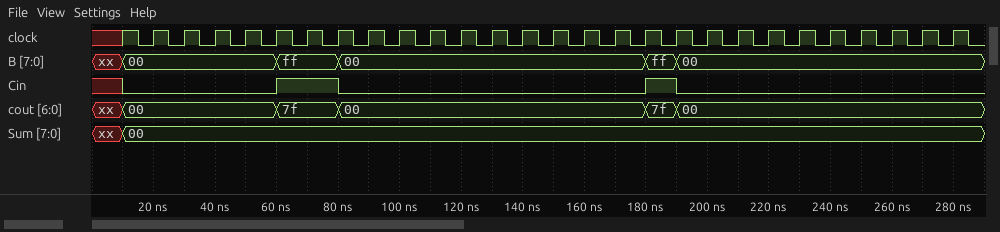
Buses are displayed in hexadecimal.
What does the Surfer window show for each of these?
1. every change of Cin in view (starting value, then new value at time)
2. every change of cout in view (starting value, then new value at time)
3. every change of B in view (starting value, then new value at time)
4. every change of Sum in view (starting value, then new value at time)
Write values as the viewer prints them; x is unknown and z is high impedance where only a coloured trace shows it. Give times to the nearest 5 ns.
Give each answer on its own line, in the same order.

x, 0 at 10 ns, 1 at 60 ns, 0 at 80 ns, 1 at 180 ns, 0 at 190 ns
xx, 00 at 10 ns, 7f at 60 ns, 00 at 80 ns, 7f at 180 ns, 00 at 190 ns
xx, 00 at 10 ns, ff at 60 ns, 00 at 80 ns, ff at 180 ns, 00 at 190 ns
xx, 00 at 10 ns
